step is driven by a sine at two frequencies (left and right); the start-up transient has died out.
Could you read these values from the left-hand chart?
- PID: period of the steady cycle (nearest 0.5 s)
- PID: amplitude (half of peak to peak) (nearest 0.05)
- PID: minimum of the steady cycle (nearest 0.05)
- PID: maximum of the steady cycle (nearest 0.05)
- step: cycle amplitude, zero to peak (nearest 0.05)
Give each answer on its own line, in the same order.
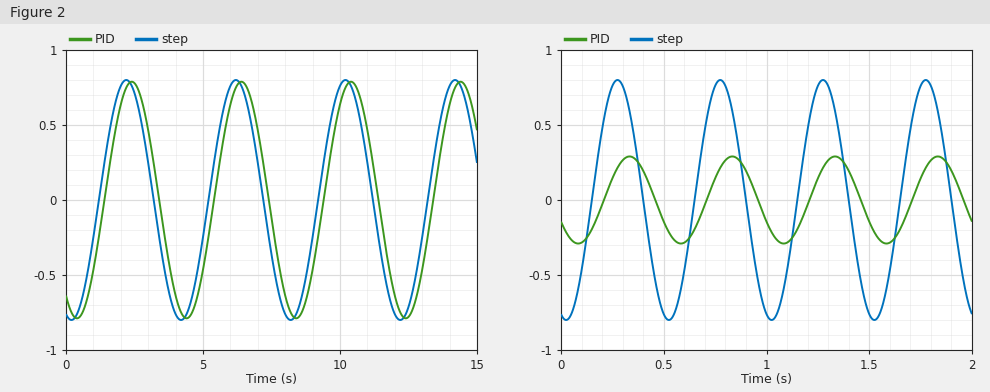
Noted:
4.0 s
0.80
-0.80
0.80
0.80
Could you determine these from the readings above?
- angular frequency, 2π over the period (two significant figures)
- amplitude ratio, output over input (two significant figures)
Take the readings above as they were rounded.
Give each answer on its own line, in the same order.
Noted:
1.6 rad/s
1.0
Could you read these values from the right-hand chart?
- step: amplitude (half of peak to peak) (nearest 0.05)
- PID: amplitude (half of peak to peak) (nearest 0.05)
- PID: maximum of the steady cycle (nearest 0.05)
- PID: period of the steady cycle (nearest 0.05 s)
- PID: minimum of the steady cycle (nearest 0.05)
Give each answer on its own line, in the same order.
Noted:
0.80
0.30
0.30
0.50 s
-0.30
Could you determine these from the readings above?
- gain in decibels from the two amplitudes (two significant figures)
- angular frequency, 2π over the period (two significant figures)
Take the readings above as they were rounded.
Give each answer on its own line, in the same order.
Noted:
-8.5 dB
13 rad/s
